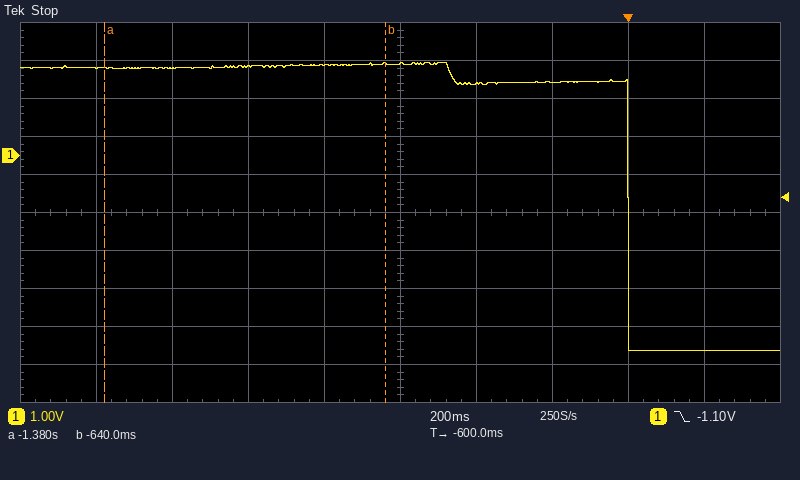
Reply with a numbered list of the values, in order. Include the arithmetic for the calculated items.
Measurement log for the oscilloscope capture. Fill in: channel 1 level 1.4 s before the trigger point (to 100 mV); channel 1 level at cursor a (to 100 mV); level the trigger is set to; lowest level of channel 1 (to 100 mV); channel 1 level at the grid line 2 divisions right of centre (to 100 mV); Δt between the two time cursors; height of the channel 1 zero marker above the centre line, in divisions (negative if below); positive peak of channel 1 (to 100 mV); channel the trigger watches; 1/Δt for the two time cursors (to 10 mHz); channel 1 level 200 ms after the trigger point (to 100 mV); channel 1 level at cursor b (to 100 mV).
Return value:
1. 2.3 V
2. 2.3 V
3. -1.10 V
4. -5.1 V
5. 1.9 V
6. -640 ms − (-1.38 s) = 740 ms
7. +1.5 div
8. 2.4 V
9. channel 1
10. 1 / 740 ms ≈ 1.35 Hz
11. -5.1 V
12. 2.4 V
